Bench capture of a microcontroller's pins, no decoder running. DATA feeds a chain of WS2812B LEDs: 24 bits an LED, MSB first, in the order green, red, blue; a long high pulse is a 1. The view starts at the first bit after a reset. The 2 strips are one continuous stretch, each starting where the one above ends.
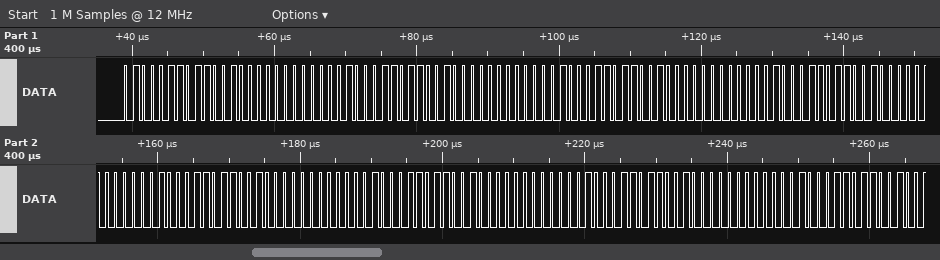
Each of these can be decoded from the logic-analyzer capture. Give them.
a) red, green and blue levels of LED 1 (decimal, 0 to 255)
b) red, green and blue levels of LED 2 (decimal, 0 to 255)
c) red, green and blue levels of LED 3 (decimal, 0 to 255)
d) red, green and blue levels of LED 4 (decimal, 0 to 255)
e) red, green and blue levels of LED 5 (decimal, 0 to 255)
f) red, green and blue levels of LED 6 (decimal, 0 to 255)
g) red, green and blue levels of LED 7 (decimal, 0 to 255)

200, 70, 0
200, 70, 0
200, 70, 0
200, 70, 0
200, 70, 0
200, 70, 0
200, 70, 0
